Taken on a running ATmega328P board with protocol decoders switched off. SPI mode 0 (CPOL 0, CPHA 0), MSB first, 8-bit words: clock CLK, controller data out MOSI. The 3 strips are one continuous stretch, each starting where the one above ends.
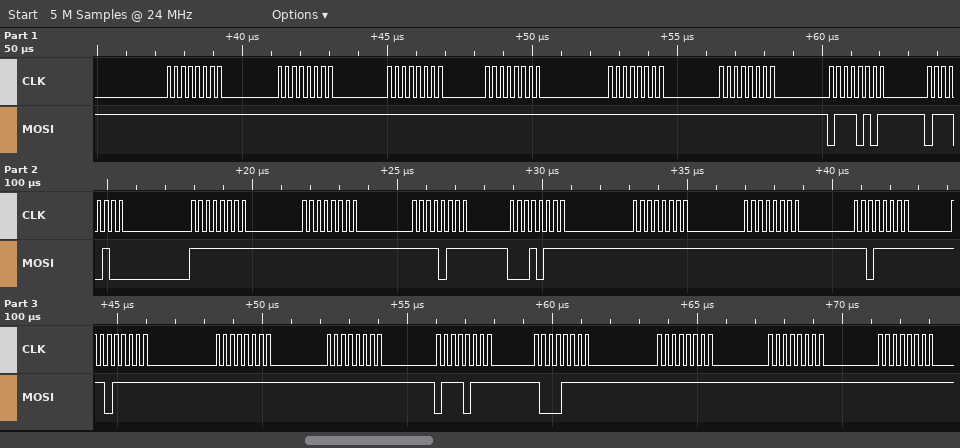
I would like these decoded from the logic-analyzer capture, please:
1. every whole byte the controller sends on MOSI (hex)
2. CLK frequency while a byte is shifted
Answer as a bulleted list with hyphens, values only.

- FF FF FF FF FF FF 75 74 FF FF F7 17 FF FF DF DF FF FF 77 8F FF FF FF
- 4 MHz
